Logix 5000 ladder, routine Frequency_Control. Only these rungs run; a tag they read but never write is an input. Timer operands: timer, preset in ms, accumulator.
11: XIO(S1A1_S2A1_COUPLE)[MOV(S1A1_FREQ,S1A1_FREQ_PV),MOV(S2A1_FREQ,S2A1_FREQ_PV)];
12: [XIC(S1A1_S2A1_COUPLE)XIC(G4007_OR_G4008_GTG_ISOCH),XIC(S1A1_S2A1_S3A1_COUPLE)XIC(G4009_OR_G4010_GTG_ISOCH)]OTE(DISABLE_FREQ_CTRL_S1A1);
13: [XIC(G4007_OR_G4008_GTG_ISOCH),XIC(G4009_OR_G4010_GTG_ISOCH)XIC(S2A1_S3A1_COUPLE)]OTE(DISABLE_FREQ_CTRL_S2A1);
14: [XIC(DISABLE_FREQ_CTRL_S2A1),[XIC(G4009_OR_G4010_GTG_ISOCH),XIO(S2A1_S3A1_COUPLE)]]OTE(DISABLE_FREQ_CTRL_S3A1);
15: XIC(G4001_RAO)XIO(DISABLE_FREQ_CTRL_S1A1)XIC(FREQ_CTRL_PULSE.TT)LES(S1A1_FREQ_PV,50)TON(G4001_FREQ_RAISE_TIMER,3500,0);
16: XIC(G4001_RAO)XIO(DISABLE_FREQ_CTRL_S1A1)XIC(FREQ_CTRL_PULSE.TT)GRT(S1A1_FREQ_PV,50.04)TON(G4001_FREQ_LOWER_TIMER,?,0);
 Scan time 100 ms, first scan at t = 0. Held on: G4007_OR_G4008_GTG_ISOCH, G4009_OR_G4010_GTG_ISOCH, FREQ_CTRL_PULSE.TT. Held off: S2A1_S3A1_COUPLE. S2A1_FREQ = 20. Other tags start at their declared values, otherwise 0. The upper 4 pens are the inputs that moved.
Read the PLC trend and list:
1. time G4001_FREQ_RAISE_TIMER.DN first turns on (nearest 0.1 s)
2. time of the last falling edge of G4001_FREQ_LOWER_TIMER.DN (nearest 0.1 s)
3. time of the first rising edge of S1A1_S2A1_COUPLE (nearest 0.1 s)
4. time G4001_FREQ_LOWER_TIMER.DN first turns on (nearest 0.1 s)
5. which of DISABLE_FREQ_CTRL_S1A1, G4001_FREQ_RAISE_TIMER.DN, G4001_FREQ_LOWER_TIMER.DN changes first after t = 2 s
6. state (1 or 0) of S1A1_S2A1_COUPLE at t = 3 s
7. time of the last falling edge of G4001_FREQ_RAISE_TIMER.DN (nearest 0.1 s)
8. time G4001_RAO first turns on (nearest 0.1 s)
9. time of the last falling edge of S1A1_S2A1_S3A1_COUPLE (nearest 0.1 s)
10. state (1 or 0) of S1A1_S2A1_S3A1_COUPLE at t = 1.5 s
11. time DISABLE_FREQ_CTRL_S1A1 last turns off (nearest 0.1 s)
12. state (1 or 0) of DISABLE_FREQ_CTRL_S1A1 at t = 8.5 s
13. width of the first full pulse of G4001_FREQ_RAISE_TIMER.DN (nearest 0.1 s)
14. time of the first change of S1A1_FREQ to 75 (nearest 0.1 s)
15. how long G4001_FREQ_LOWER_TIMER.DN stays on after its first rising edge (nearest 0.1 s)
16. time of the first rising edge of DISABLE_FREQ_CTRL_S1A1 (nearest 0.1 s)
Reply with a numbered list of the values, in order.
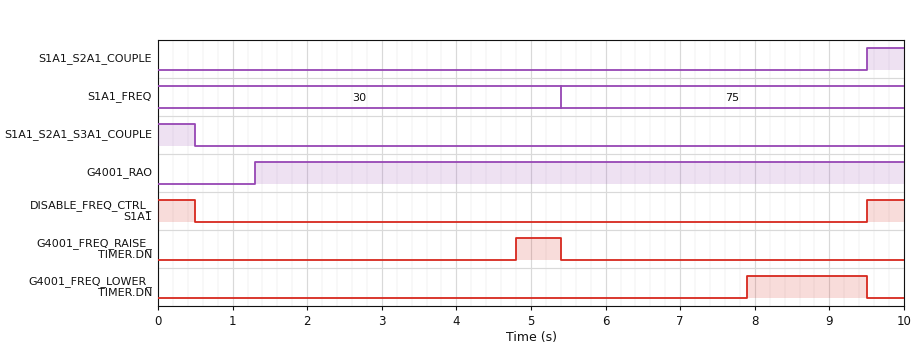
1. 4.8 s
2. 9.5 s
3. 9.5 s
4. 7.9 s
5. G4001_FREQ_RAISE_TIMER.DN
6. 0
7. 5.4 s
8. 1.3 s
9. 0.5 s
10. 0
11. 0.5 s
12. 0
13. 0.6 s
14. 5.4 s
15. 1.6 s
16. 9.5 s
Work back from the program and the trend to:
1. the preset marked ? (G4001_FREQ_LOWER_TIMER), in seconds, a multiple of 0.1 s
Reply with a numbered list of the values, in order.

1. 2.5 s
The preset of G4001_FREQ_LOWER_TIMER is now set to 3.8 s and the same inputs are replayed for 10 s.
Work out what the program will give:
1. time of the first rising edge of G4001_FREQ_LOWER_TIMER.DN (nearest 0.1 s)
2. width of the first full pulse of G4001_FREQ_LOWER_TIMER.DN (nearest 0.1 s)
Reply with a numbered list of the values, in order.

1. 9.2 s
2. 0.3 s
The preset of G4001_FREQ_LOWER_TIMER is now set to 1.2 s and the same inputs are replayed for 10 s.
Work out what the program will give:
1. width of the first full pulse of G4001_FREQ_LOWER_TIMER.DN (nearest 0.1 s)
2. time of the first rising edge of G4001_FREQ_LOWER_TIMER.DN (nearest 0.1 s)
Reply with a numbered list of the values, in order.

1. 2.9 s
2. 6.6 s
